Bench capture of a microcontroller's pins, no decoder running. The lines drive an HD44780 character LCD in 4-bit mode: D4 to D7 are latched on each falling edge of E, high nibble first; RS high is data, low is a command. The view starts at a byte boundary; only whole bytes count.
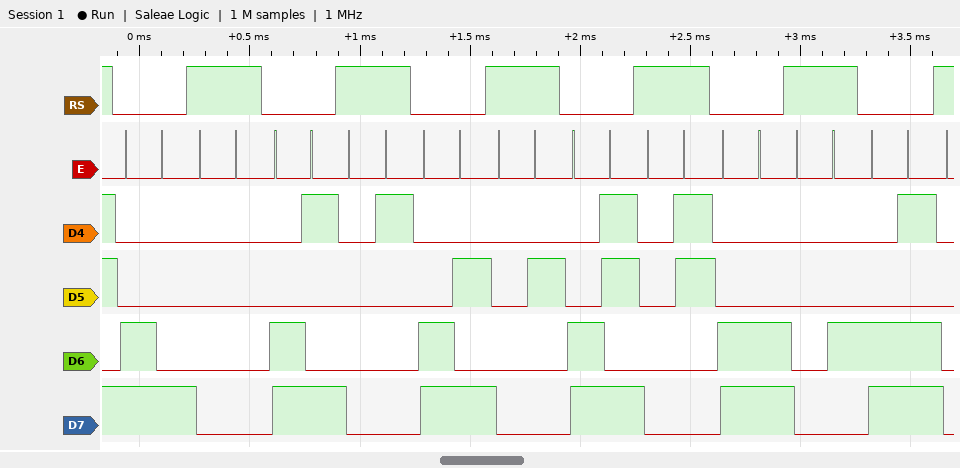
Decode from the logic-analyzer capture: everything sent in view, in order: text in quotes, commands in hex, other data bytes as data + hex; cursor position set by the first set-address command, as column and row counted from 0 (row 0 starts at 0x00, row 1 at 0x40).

0xC8 data 00 0xC9 data 01 0xCA data 02 0xCB data 03 0xCC data 04 0xCD
column 8, row 1
